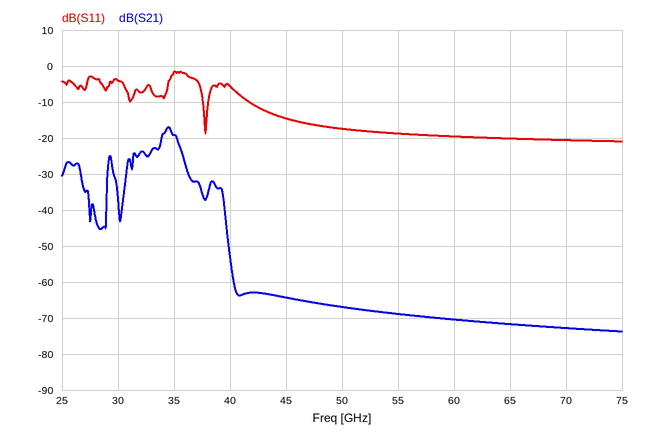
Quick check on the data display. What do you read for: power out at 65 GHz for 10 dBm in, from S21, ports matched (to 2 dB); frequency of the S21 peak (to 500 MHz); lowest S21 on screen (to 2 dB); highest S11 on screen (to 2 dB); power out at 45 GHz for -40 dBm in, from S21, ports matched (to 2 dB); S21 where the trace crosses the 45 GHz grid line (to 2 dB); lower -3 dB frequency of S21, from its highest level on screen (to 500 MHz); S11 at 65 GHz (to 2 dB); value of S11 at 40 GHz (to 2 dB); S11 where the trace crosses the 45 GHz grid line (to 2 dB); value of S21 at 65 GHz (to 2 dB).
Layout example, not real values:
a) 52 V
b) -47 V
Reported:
a) -62 dBm
b) 34.5 GHz
c) -74 dB
d) -2 dB
e) -104 dBm
f) -64 dB
g) 34.0 GHz
h) -20 dB
i) -6 dB
j) -14 dB
k) -72 dB
